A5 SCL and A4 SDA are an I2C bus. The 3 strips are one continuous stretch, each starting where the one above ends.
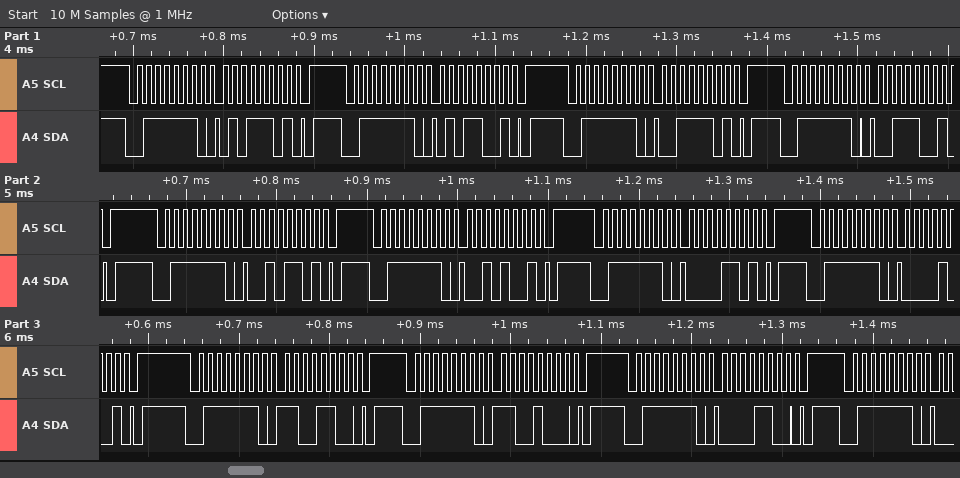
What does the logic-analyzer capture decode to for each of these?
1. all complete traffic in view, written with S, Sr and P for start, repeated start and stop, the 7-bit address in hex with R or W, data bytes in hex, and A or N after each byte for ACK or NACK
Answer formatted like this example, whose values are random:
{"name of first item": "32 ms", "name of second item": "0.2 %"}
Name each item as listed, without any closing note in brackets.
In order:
{"all complete traffic in view, written with S, Sr and P for start, repeated start and stop, the 7-bit address in hex with R or W, data bytes in hex, and A or N after each byte for ACK or NACK": "S 3FW A 5D A P S 3FW A 59 A P S 3FW A 3D A P S 3FW A 39 A P S 3FW A 2D A P S 3FW A 29 A P S 3FW A 0D A P S 3FW A 09 A P S 3FW A CC A P S 3FW A C8 A P S 3FW A 0C A P S 3FW A"}
